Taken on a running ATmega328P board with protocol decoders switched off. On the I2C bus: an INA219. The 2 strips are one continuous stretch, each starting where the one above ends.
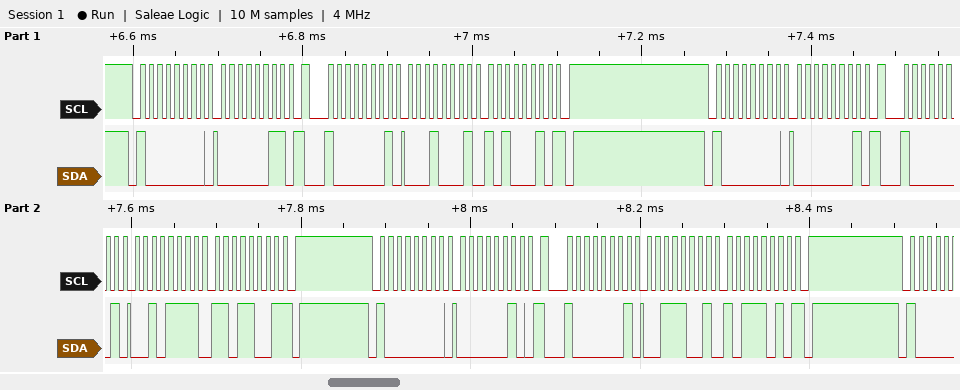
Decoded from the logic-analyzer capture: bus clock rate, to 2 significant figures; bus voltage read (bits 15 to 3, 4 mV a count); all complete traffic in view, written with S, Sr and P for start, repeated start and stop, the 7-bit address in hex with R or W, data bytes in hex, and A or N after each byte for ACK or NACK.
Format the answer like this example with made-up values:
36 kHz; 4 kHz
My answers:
100 kHz; 7.388 V; S 40W A 03 A Sr 40R A 11 A A2 N P S 40W A 01 A Sr 40R A 2F A D9 N P S 40W A 02 A Sr 40R A 39 A BA N P
